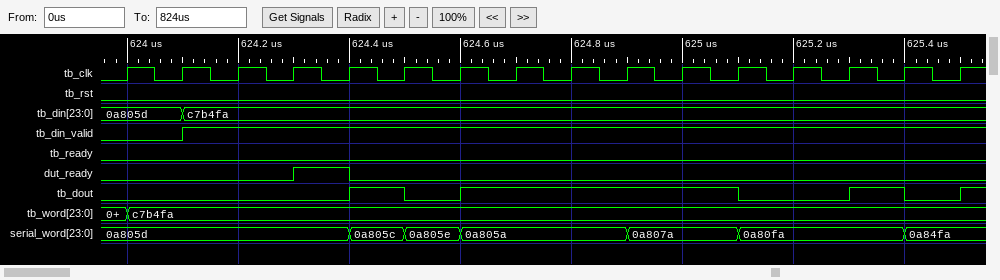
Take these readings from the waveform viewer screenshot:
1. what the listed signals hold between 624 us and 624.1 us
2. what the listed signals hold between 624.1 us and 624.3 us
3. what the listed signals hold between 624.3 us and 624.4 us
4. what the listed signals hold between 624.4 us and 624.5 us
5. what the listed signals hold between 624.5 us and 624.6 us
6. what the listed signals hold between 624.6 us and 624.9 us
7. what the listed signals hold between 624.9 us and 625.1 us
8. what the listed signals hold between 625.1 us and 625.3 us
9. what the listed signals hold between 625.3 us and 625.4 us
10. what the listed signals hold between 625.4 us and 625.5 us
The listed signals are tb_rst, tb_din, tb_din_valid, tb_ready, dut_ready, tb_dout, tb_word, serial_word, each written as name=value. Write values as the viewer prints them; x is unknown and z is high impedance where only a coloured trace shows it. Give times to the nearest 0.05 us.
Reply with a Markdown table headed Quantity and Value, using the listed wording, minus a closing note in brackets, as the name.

| Quantity | Value |
|---|---|
| what the listed signals hold between 624 us and 624.1 us | tb_rst=0, tb_din=0a805d, tb_din_valid=0, tb_ready=0, dut_ready=0, tb_dout=0, tb_word=c7b4fa, serial_word=0a805d |
| what the listed signals hold between 624.1 us and 624.3 us | tb_rst=0, tb_din=c7b4fa, tb_din_valid=1, tb_ready=0, dut_ready=0, tb_dout=0, tb_word=c7b4fa, serial_word=0a805d |
| what the listed signals hold between 624.3 us and 624.4 us | tb_rst=0, tb_din=c7b4fa, tb_din_valid=1, tb_ready=0, dut_ready=1, tb_dout=0, tb_word=c7b4fa, serial_word=0a805d |
| what the listed signals hold between 624.4 us and 624.5 us | tb_rst=0, tb_din=c7b4fa, tb_din_valid=1, tb_ready=0, dut_ready=0, tb_dout=1, tb_word=c7b4fa, serial_word=0a805c |
| what the listed signals hold between 624.5 us and 624.6 us | tb_rst=0, tb_din=c7b4fa, tb_din_valid=1, tb_ready=0, dut_ready=0, tb_dout=0, tb_word=c7b4fa, serial_word=0a805e |
| what the listed signals hold between 624.6 us and 624.9 us | tb_rst=0, tb_din=c7b4fa, tb_din_valid=1, tb_ready=0, dut_ready=0, tb_dout=1, tb_word=c7b4fa, serial_word=0a805a |
| what the listed signals hold between 624.9 us and 625.1 us | tb_rst=0, tb_din=c7b4fa, tb_din_valid=1, tb_ready=0, dut_ready=0, tb_dout=1, tb_word=c7b4fa, serial_word=0a807a |
| what the listed signals hold between 625.1 us and 625.3 us | tb_rst=0, tb_din=c7b4fa, tb_din_valid=1, tb_ready=0, dut_ready=0, tb_dout=0, tb_word=c7b4fa, serial_word=0a80fa |
| what the listed signals hold between 625.3 us and 625.4 us | tb_rst=0, tb_din=c7b4fa, tb_din_valid=1, tb_ready=0, dut_ready=0, tb_dout=1, tb_word=c7b4fa, serial_word=0a80fa |
| what the listed signals hold between 625.4 us and 625.5 us | tb_rst=0, tb_din=c7b4fa, tb_din_valid=1, tb_ready=0, dut_ready=0, tb_dout=0, tb_word=c7b4fa, serial_word=0a84fa |
